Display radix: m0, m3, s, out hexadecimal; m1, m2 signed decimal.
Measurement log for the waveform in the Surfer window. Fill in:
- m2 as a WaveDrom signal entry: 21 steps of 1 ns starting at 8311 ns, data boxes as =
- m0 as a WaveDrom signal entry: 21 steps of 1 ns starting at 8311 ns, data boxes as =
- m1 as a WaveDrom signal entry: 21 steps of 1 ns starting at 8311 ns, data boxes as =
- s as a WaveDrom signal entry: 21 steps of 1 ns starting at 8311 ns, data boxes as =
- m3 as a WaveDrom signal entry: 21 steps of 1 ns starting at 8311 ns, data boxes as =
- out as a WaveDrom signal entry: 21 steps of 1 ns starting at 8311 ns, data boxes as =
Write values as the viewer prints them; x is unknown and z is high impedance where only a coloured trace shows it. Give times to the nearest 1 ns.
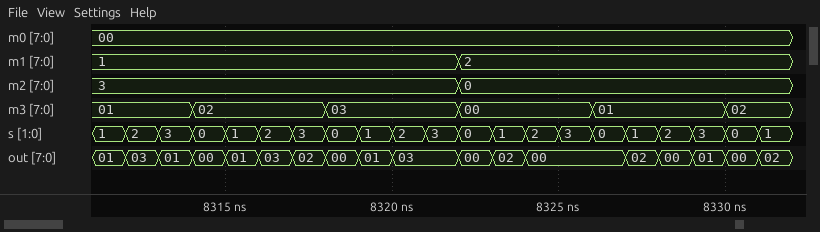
{name: 'm2', wave: '=..........=.........', data: '3 0'}
{name: 'm0', wave: '=....................', data: '00'}
{name: 'm1', wave: '=..........=.........', data: '1 2'}
{name: 's', wave: '=====================', data: '1 2 3 0 1 2 3 0 1 2 3 0 1 2 3 0 1 2 3 0 1'}
{name: 'm3', wave: '=..=...=...=...=...=.', data: '01 02 03 00 01 02'}
{name: 'out', wave: '==========.===..=====', data: '01 03 01 00 01 03 02 00 01 03 00 02 00 02 00 01 00 02'}
